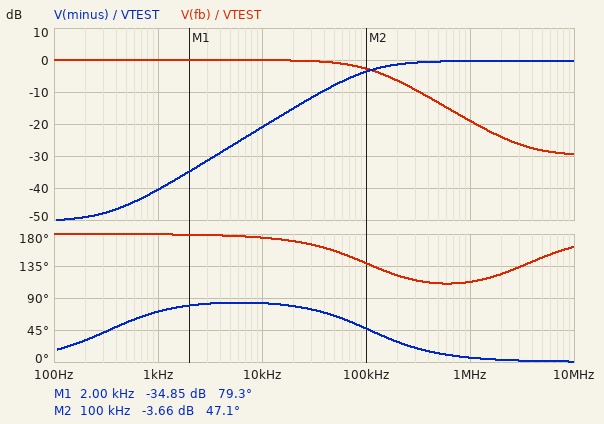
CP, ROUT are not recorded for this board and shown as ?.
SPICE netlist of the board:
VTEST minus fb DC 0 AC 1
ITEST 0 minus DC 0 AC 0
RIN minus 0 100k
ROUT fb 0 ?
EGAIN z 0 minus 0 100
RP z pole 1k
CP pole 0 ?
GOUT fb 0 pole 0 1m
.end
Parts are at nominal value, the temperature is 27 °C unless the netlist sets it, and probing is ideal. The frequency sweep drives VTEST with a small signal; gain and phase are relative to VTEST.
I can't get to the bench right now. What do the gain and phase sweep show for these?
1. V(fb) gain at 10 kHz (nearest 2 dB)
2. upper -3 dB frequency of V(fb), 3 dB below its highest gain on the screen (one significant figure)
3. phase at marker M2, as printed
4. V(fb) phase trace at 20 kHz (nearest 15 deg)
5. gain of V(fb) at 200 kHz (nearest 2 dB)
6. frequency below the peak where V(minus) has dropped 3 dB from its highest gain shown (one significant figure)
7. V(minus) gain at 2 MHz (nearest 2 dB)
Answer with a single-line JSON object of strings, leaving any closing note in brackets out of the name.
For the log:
{"V(fb) gain at 10 kHz": "0 dB", "upper -3 dB frequency of V(fb), 3 dB below its highest gain on the screen": "100 kHz", "phase at marker M2, as printed": "47.1 deg", "V(fb) phase trace at 20 kHz": "165 deg", "gain of V(fb) at 200 kHz": "-6 dB", "frequency below the peak where V(minus) has dropped 3 dB from its highest gain shown": "100 kHz", "V(minus) gain at 2 MHz": "0 dB"}
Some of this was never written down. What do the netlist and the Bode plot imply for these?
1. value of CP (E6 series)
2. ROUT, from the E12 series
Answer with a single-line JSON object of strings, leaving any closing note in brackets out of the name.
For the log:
{"value of CP": "470 nF", "ROUT, from the E12 series": "3.3 kΩ"}
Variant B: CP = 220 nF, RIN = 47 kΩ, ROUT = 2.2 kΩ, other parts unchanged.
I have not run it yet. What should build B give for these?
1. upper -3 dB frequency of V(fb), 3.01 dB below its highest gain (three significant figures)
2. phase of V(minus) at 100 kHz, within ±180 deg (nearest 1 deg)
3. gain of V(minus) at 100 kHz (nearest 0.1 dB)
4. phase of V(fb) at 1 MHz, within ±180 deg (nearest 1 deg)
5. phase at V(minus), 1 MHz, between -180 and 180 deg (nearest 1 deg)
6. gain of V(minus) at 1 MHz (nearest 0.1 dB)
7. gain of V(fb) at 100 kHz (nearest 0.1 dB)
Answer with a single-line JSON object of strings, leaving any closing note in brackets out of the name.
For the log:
{"upper -3 dB frequency of V(fb), 3.01 dB below its highest gain": "153 kHz", "phase of V(minus) at 100 kHz, within ±180 deg": "56 deg", "gain of V(minus) at 100 kHz": "-5.6 dB", "phase of V(fb) at 1 MHz, within ±180 deg": "115 deg", "phase at V(minus), 1 MHz, between -180 and 180 deg": "9 deg", "gain of V(minus) at 1 MHz": "-0.5 dB", "gain of V(fb) at 100 kHz": "-1.6 dB"}
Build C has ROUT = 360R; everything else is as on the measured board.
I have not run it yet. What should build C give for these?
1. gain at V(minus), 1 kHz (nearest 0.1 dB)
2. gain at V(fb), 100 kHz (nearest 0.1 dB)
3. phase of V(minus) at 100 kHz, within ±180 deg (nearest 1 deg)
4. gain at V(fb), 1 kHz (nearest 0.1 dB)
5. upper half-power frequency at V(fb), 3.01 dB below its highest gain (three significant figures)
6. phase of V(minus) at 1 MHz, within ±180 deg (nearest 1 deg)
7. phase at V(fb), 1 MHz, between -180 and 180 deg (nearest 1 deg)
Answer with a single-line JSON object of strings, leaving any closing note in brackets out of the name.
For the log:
{"gain at V(minus), 1 kHz": "-21.5 dB", "gain at V(fb), 100 kHz": "-18.4 dB", "phase of V(minus) at 100 kHz, within ±180 deg": "7 deg", "gain at V(fb), 1 kHz": "-0.3 dB", "upper half-power frequency at V(fb), 3.01 dB below its highest gain": "12.5 kHz", "phase of V(minus) at 1 MHz, within ±180 deg": "1 deg", "phase at V(fb), 1 MHz, between -180 and 180 deg": "107 deg"}
